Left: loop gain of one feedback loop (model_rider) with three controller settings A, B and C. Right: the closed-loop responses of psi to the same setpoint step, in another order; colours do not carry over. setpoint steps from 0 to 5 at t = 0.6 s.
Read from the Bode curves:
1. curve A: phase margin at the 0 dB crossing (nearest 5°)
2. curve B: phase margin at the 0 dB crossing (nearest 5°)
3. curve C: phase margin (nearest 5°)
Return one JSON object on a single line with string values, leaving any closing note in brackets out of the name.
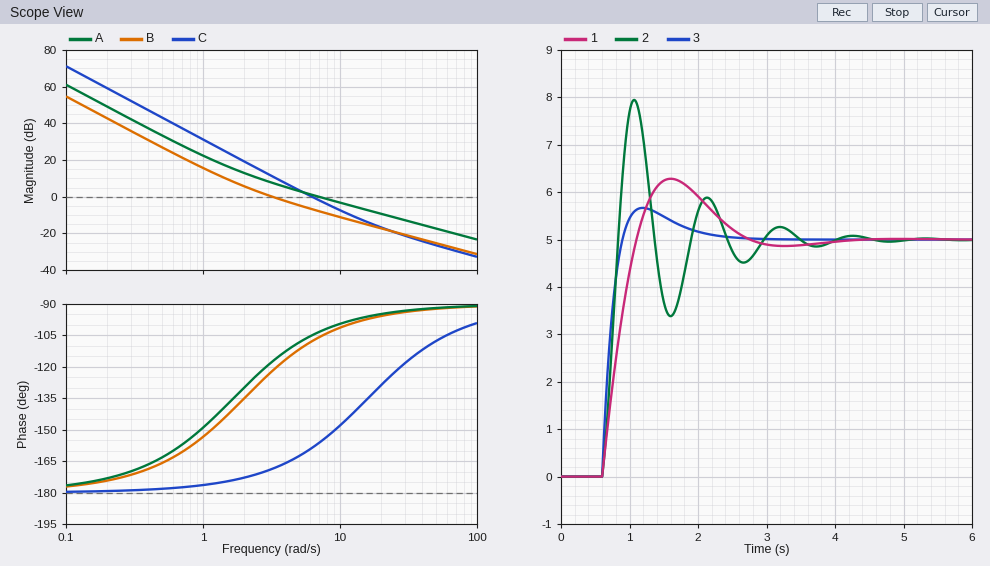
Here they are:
{"curve A: phase margin at the 0 dB crossing": "75°", "curve B: phase margin at the 0 dB crossing": "60°", "curve C: phase margin": "20°"}
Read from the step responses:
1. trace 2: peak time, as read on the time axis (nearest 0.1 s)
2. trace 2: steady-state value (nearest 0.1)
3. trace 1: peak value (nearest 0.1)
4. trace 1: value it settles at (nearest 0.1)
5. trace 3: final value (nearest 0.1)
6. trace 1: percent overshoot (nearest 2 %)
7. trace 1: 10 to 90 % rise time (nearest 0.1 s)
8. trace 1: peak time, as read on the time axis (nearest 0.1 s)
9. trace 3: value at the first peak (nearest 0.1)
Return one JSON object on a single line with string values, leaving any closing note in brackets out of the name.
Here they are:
{"trace 2: peak time, as read on the time axis": "1.1 s", "trace 2: steady-state value": "5.0", "trace 1: peak value": "6.3", "trace 1: value it settles at": "5.0", "trace 3: final value": "5.0", "trace 1: percent overshoot": "26 %", "trace 1: 10 to 90 % rise time": "0.4 s", "trace 1: peak time, as read on the time axis": "1.6 s", "trace 3: value at the first peak": "5.7"}
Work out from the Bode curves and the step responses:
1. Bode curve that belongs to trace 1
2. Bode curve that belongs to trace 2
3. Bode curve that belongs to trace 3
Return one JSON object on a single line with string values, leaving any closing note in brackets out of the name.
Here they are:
{"Bode curve that belongs to trace 1": "B", "Bode curve that belongs to trace 2": "C", "Bode curve that belongs to trace 3": "A"}
